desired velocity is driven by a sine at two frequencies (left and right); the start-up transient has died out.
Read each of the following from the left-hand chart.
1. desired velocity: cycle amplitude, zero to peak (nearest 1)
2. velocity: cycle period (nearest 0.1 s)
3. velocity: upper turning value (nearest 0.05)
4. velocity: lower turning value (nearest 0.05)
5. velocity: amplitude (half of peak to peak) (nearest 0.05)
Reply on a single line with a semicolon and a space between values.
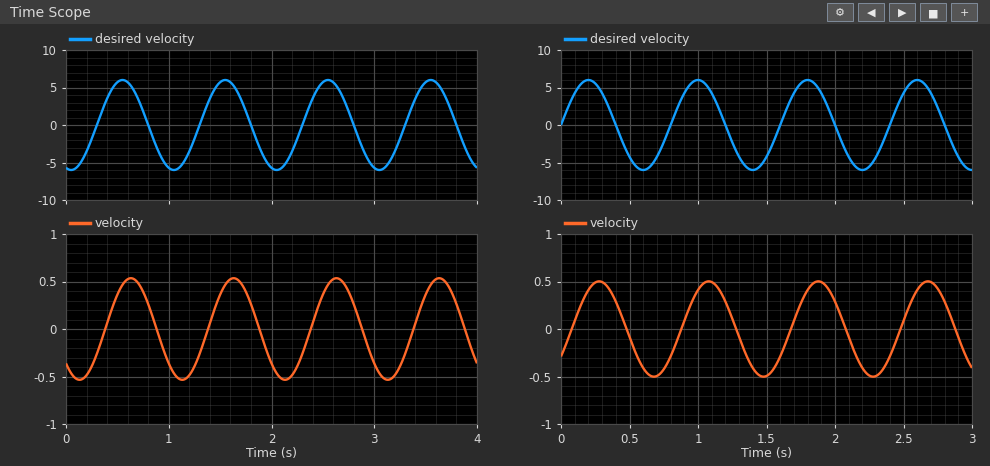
6; 1.0 s; 0.55; -0.55; 0.55
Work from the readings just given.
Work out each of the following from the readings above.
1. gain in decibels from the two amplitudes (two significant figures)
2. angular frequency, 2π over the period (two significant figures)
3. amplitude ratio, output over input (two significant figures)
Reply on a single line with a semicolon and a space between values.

-21 dB; 6.3 rad/s; 0.092
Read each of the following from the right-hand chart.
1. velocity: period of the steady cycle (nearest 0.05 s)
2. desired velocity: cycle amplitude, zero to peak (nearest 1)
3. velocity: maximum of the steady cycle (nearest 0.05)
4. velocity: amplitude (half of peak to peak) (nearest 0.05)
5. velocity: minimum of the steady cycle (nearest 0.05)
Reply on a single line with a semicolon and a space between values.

0.80 s; 6; 0.50; 0.50; -0.50
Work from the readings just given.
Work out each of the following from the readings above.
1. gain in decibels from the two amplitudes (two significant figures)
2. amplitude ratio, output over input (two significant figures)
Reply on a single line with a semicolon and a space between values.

-22 dB; 0.083
